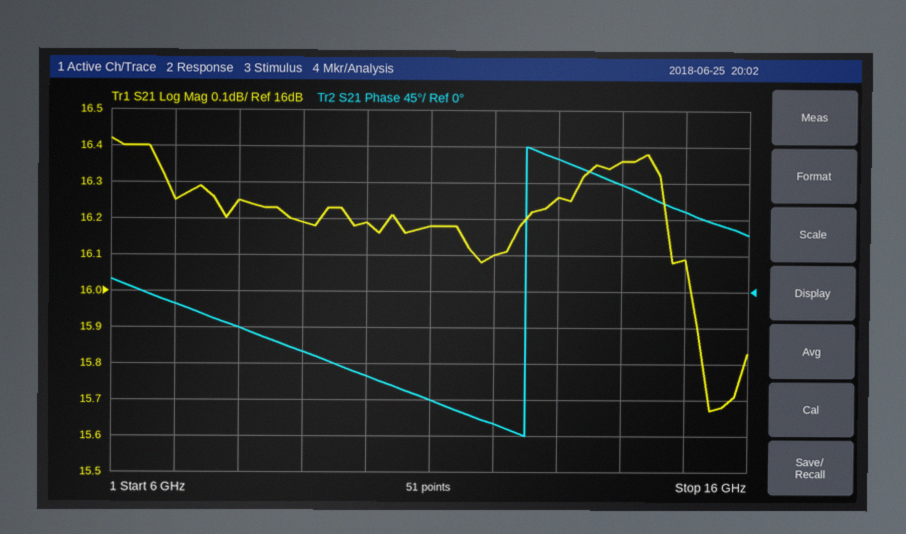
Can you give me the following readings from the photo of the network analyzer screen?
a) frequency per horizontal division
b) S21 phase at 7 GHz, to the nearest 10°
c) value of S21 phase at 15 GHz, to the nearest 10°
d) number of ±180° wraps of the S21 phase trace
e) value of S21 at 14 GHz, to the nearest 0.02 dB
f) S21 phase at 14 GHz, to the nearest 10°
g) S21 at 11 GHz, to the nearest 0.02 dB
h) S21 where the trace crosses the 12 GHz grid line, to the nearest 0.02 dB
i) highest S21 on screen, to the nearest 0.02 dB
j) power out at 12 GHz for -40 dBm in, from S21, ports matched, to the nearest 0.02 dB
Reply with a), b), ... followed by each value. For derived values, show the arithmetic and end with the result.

a) 1 GHz
b) -20°
c) 100°
d) 1
e) 16.36 dB
f) 130°
g) 16.18 dB
h) 16.10 dB
i) 16.42 dB
j) -40 dBm + (16.10 dB) = -23.90 dBm
